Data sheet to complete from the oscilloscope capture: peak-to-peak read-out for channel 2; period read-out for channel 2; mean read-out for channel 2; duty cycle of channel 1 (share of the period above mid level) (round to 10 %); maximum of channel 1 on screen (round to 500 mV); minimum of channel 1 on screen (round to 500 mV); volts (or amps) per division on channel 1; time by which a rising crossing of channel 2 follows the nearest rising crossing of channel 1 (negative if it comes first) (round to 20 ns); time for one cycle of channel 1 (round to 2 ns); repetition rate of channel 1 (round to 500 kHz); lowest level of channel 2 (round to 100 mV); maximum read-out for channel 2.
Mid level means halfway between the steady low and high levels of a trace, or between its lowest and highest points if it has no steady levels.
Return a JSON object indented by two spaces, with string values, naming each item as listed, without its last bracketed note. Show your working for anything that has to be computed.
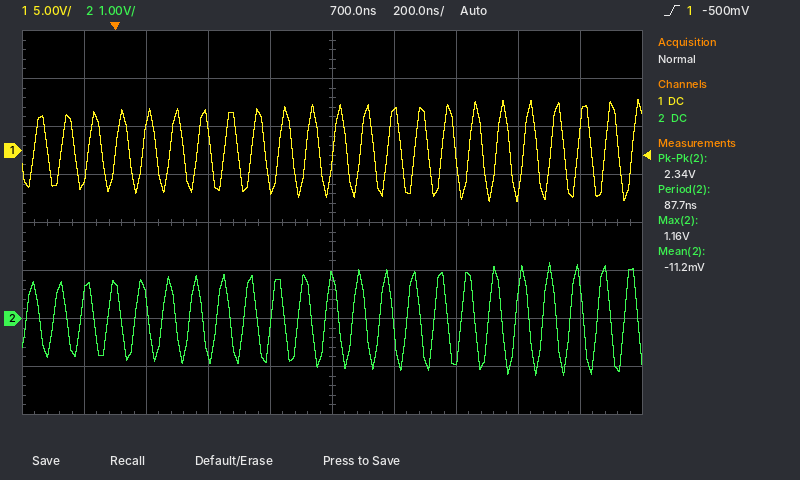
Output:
{
  "peak-to-peak read-out for channel 2": "2.34 V",
  "period read-out for channel 2": "87.7 ns",
  "mean read-out for channel 2": "-11.2 mV",
  "duty cycle of channel 1 (share of the period above mid level)": "50 %",
  "maximum of channel 1 on screen": "5.5 V",
  "minimum of channel 1 on screen": "-5.5 V",
  "volts (or amps) per division on channel 1": "5 V",
  "time by which a rising crossing of channel 2 follows the nearest rising crossing of channel 1 (negative if it comes first)": "-20 ns",
  "time for one cycle of channel 1": "88 ns",
  "repetition rate of channel 1": "1 / 88 ns ≈ 11.4 MHz, so 11.5 MHz to the nearest 500 kHz",
  "lowest level of channel 2": "-1.2 V",
  "maximum read-out for channel 2": "1.16 V"
}
